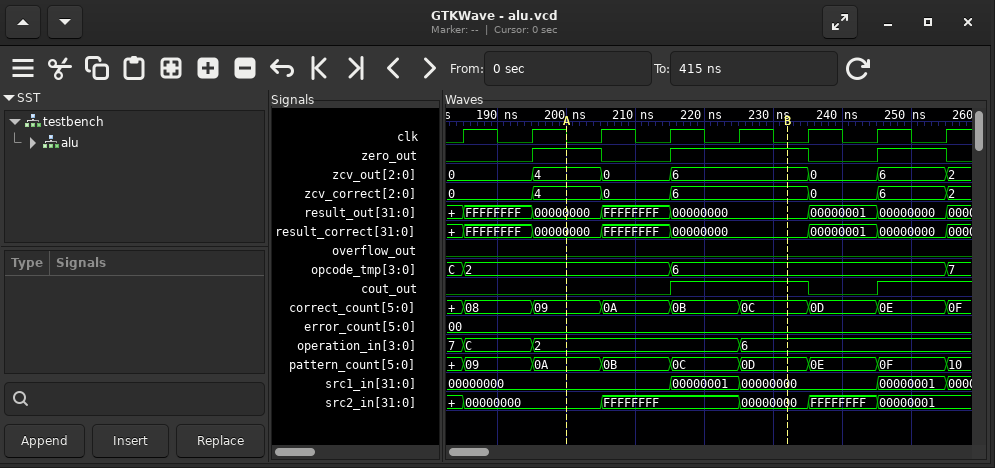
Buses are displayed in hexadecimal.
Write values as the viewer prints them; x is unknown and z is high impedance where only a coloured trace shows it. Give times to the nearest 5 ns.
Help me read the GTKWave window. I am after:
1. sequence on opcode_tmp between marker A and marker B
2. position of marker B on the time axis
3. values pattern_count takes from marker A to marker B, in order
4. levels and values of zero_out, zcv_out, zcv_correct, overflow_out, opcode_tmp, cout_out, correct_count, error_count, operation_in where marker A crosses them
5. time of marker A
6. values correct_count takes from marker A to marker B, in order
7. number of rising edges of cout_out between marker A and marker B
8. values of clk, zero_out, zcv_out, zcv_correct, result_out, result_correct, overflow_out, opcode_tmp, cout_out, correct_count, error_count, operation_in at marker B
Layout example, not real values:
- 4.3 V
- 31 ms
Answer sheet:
- 2, 6
- 230 ns
- 0A, 0B, 0C, 0D
- zero_out=1, zcv_out=4, zcv_correct=4, overflow_out=0, opcode_tmp=2, cout_out=0, correct_count=09, error_count=00, operation_in=2
- 200 ns
- 09, 0A, 0B, 0C
- 1
- clk=0, zero_out=1, zcv_out=6, zcv_correct=6, result_out=00000000, result_correct=00000000, overflow_out=0, opcode_tmp=6, cout_out=1, correct_count=0C, error_count=00, operation_in=6
